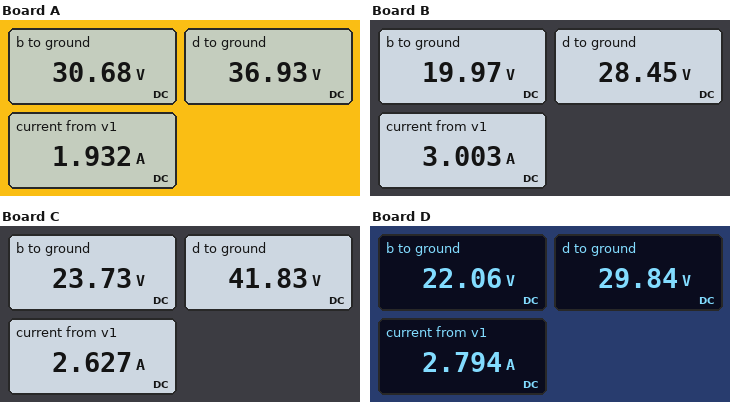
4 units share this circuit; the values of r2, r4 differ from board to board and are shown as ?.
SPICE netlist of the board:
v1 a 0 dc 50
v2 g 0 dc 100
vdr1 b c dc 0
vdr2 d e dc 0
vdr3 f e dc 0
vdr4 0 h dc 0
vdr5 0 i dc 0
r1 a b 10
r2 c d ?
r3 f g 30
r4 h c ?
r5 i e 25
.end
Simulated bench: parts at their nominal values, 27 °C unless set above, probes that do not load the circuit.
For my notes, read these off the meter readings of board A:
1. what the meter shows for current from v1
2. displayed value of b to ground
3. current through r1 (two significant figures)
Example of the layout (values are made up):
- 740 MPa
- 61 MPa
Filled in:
- 1.932 A
- 30.68 V
- 1.9 A
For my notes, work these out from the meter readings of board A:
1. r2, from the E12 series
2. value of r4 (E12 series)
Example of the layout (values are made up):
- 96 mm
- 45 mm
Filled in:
- 10 Ω
- 12 Ω
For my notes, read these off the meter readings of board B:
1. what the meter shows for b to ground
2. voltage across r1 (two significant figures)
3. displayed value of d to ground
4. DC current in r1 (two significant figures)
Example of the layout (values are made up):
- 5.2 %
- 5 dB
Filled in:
- 19.97 V
- 30 V
- 28.45 V
- 3.0 A
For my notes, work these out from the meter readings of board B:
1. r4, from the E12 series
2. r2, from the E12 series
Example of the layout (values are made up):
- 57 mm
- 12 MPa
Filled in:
- 4.7 Ω
- 6.8 Ω
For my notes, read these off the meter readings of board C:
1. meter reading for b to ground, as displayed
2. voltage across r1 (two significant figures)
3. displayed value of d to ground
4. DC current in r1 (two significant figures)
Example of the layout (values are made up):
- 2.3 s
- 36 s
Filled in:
- 23.73 V
- 26 V
- 41.83 V
- 2.6 A
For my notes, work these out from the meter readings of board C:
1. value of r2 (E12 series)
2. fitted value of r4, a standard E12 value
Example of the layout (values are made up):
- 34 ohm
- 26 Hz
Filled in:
- 68 Ω
- 8.2 Ω
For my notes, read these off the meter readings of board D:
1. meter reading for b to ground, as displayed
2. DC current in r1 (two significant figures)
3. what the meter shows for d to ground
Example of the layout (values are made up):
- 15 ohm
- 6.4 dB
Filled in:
- 22.06 V
- 2.8 A
- 29.84 V
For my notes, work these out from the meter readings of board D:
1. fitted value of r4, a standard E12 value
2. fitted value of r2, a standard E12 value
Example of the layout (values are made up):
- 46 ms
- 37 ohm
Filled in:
- 5.6 Ω
- 6.8 Ω
